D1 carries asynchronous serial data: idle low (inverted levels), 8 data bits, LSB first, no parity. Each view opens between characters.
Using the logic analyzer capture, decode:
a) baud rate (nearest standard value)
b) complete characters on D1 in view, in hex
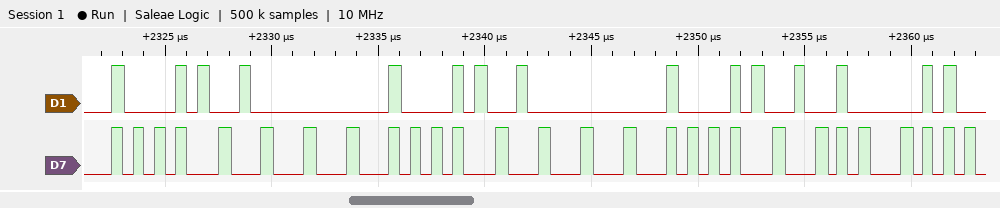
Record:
2000000 baud
5F, FF, 5F, FF, 5F, F7
